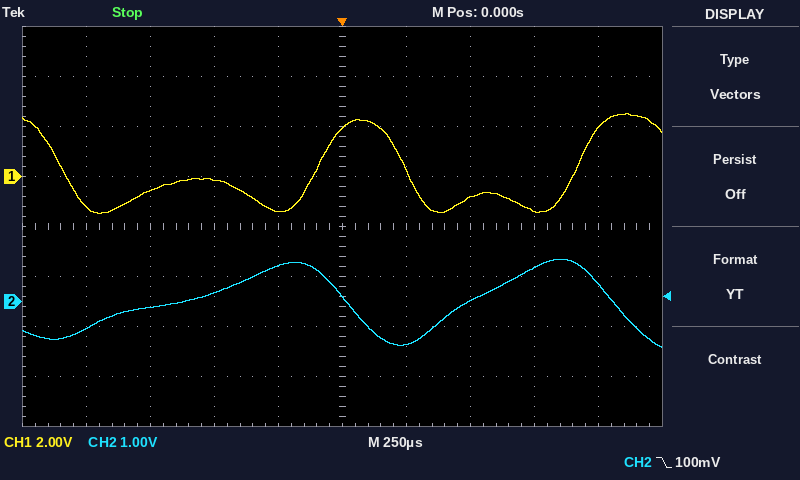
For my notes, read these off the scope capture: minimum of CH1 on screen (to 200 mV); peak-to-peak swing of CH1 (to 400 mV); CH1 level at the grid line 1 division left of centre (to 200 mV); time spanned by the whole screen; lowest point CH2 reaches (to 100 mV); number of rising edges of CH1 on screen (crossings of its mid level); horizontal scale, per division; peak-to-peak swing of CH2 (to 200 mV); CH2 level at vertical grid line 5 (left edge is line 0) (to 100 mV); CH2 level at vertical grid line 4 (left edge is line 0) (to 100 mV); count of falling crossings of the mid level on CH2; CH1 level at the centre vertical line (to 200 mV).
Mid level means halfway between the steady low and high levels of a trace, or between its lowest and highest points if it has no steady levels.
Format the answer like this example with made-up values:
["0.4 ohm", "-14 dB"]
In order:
["-1.4 V", "4.0 V", "-1.4 V", "2.5 ms", "-900 mV", "2", "250 µs", "1.8 V", "100 mV", "700 mV", "2", "2.0 V"]
